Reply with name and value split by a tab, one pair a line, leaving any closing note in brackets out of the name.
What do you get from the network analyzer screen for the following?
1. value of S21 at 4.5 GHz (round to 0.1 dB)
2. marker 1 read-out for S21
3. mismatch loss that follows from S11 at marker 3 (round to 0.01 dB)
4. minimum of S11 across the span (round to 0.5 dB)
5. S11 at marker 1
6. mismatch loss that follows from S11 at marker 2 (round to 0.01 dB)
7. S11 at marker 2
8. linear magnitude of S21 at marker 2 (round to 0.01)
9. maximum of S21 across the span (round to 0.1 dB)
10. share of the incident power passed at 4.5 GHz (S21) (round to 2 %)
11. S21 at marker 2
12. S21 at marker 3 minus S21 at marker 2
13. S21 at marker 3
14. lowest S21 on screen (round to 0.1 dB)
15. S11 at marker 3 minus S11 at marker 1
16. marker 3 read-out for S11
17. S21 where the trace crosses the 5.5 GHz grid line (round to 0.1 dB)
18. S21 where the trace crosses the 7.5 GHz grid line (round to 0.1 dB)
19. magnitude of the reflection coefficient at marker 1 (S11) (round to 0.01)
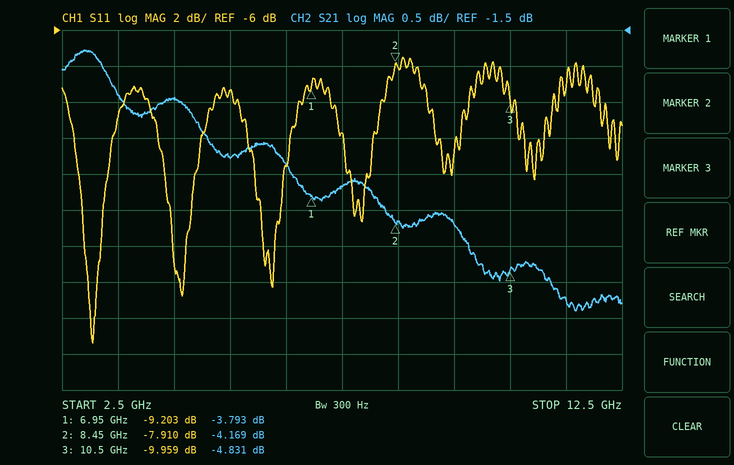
value of S21 at 4.5 GHz	-2.5 dB
marker 1 read-out for S21	-3.793 dB
mismatch loss that follows from S11 at marker 3	0.46 dB
minimum of S11 across the span	-23.5 dB
S11 at marker 1	-9.203 dB
mismatch loss that follows from S11 at marker 2	0.77 dB
S11 at marker 2	-7.910 dB
linear magnitude of S21 at marker 2	0.62
maximum of S21 across the span	-1.8 dB
share of the incident power passed at 4.5 GHz (S21)	56 %
S21 at marker 2	-4.169 dB
S21 at marker 3 minus S21 at marker 2	-0.662 dB
S21 at marker 3	-4.831 dB
lowest S21 on screen	-5.4 dB
S11 at marker 3 minus S11 at marker 1	-0.756 dB
marker 3 read-out for S11	-9.959 dB
S21 where the trace crosses the 5.5 GHz grid line	-3.3 dB
S21 where the trace crosses the 7.5 GHz grid line	-3.7 dB
magnitude of the reflection coefficient at marker 1 (S11)	0.35
